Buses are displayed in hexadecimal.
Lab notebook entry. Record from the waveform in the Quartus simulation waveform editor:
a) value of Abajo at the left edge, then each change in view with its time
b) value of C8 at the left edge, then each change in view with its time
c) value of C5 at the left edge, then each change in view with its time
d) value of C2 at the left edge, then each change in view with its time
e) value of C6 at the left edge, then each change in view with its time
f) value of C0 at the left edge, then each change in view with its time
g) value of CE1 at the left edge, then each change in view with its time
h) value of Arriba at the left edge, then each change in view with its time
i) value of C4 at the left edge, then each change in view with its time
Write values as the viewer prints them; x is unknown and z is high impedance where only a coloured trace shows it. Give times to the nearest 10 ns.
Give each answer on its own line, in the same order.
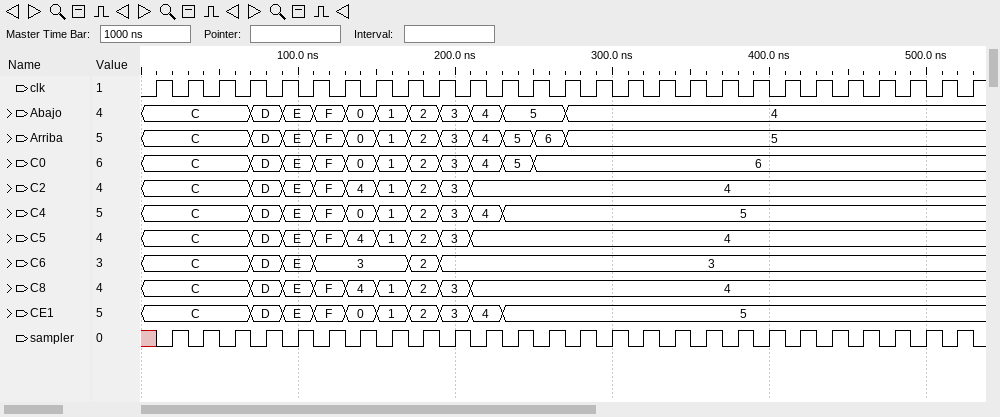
C, D at 70 ns, E at 90 ns, F at 110 ns, 0 at 130 ns, 1 at 150 ns, 2 at 170 ns, 3 at 190 ns, 4 at 210 ns, 5 at 230 ns, 4 at 270 ns
C, D at 70 ns, E at 90 ns, F at 110 ns, 4 at 130 ns, 1 at 150 ns, 2 at 170 ns, 3 at 190 ns, 4 at 210 ns
C, D at 70 ns, E at 90 ns, F at 110 ns, 4 at 130 ns, 1 at 150 ns, 2 at 170 ns, 3 at 190 ns, 4 at 210 ns
C, D at 70 ns, E at 90 ns, F at 110 ns, 4 at 130 ns, 1 at 150 ns, 2 at 170 ns, 3 at 190 ns, 4 at 210 ns
C, D at 70 ns, E at 90 ns, 3 at 110 ns, 2 at 170 ns, 3 at 190 ns
C, D at 70 ns, E at 90 ns, F at 110 ns, 0 at 130 ns, 1 at 150 ns, 2 at 170 ns, 3 at 190 ns, 4 at 210 ns, 5 at 230 ns, 6 at 250 ns
C, D at 70 ns, E at 90 ns, F at 110 ns, 0 at 130 ns, 1 at 150 ns, 2 at 170 ns, 3 at 190 ns, 4 at 210 ns, 5 at 230 ns
C, D at 70 ns, E at 90 ns, F at 110 ns, 0 at 130 ns, 1 at 150 ns, 2 at 170 ns, 3 at 190 ns, 4 at 210 ns, 5 at 230 ns, 6 at 250 ns, 5 at 270 ns
C, D at 70 ns, E at 90 ns, F at 110 ns, 0 at 130 ns, 1 at 150 ns, 2 at 170 ns, 3 at 190 ns, 4 at 210 ns, 5 at 230 ns
